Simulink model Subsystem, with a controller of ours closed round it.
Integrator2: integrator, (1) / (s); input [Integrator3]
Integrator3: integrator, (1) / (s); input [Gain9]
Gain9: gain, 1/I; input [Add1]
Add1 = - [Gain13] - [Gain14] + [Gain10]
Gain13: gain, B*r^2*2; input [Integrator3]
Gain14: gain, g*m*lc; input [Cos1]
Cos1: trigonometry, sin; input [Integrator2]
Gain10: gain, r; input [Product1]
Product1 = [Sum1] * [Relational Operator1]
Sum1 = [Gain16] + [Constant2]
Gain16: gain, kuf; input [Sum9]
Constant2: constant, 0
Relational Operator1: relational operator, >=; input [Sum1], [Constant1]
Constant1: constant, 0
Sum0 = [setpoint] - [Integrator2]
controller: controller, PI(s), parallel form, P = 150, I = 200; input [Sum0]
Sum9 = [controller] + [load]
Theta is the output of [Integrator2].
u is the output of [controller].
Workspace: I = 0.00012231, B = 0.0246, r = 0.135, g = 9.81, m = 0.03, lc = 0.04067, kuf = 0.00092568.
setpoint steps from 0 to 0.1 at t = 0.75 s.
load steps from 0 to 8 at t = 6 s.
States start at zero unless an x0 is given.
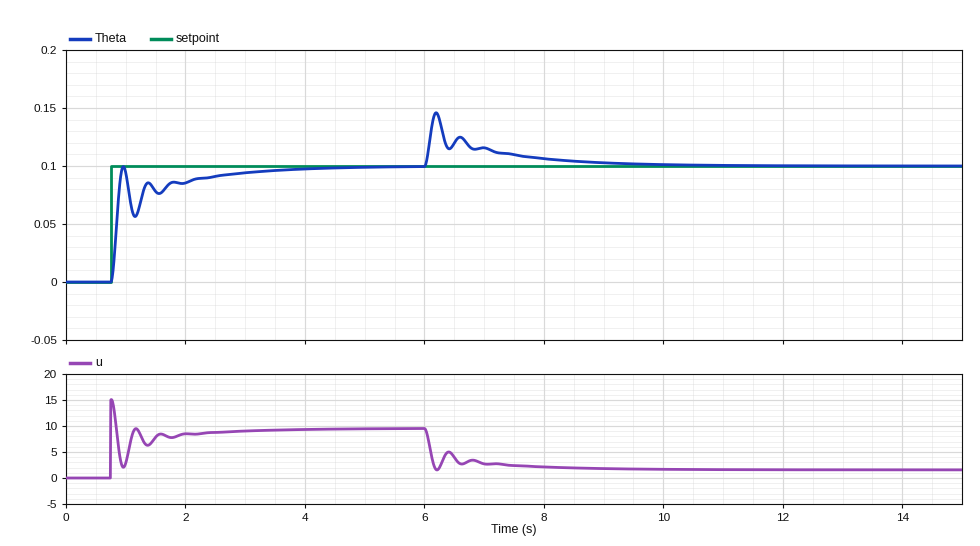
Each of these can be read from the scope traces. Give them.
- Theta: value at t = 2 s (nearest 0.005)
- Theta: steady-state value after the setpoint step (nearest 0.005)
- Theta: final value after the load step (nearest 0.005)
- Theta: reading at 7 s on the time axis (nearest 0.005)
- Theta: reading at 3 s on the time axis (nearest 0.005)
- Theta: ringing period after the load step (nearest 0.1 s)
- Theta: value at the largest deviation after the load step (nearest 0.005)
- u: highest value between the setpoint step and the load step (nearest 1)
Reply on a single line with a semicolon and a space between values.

0.085; 0.100; 0.100; 0.115; 0.095; 0.4 s; 0.145; 15
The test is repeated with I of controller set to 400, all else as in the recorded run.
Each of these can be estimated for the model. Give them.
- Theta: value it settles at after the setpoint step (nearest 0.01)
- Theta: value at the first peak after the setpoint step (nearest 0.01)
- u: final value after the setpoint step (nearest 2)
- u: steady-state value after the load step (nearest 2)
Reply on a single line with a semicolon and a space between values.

0.10; 0.11; 10; 2
